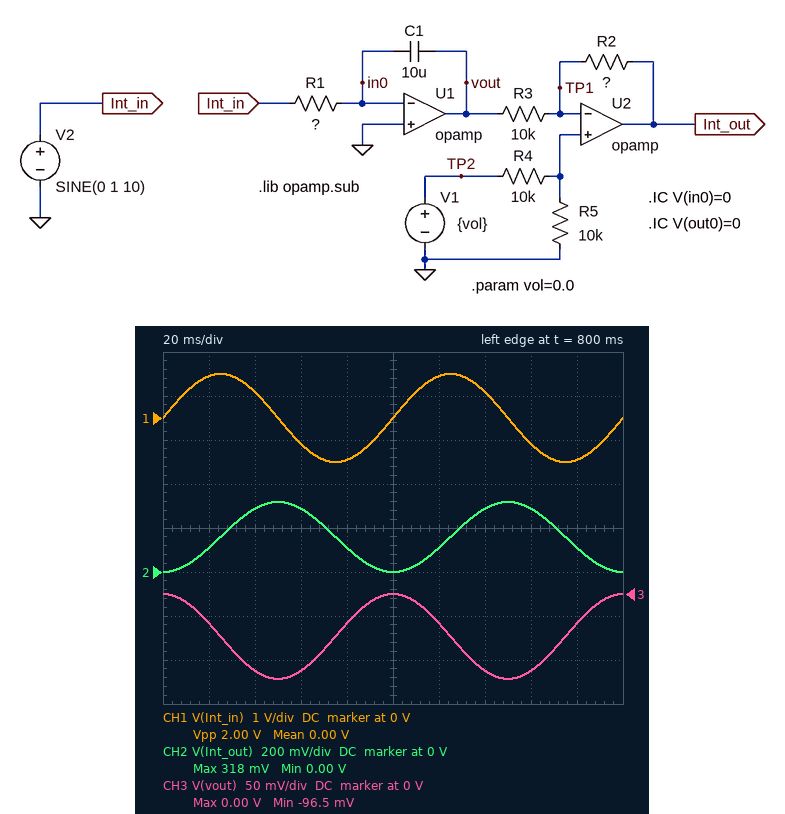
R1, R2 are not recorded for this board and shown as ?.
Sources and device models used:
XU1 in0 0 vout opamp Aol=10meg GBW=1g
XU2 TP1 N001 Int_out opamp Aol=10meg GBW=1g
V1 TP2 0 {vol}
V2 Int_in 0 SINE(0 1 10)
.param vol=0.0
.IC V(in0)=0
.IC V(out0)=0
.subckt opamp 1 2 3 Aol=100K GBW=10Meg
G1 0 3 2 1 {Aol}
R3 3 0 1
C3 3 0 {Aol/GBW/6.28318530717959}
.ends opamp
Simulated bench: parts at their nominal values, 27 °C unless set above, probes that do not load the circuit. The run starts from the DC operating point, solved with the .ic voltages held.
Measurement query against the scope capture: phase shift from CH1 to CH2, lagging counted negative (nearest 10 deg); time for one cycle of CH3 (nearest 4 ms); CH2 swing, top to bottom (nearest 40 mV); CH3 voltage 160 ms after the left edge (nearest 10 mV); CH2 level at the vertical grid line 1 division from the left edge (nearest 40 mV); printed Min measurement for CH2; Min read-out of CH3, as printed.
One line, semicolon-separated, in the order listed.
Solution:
-90 deg; 100 ms; 320 mV; -90 mV; 120 mV; 0.00 V; -96.5 mV
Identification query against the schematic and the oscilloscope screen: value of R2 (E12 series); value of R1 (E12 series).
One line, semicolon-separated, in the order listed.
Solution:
33 kΩ; 33 kΩ
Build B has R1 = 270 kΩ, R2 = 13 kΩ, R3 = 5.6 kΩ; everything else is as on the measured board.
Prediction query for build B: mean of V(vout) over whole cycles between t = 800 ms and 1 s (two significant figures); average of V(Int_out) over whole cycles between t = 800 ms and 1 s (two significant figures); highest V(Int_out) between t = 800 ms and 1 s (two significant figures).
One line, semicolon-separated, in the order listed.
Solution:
-5.9 mV; 14 mV; 27 mV
